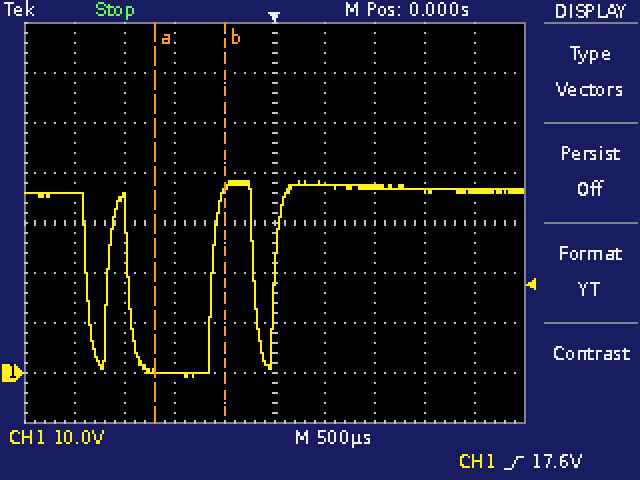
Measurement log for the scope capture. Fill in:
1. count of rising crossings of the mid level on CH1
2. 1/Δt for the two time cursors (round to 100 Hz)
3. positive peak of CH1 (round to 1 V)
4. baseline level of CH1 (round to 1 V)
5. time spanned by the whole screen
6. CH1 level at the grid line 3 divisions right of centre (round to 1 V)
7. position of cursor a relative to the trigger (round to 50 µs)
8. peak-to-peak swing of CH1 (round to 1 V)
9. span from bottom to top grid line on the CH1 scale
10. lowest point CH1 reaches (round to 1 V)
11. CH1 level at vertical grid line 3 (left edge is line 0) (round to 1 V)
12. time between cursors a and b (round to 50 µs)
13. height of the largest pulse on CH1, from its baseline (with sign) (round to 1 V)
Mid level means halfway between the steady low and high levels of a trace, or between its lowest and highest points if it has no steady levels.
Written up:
3
1.4 kHz
38 V
36 V
5 ms
36 V
-1.20 ms
39 V
80 V
-1 V
0 V
700 µs
-37 V
